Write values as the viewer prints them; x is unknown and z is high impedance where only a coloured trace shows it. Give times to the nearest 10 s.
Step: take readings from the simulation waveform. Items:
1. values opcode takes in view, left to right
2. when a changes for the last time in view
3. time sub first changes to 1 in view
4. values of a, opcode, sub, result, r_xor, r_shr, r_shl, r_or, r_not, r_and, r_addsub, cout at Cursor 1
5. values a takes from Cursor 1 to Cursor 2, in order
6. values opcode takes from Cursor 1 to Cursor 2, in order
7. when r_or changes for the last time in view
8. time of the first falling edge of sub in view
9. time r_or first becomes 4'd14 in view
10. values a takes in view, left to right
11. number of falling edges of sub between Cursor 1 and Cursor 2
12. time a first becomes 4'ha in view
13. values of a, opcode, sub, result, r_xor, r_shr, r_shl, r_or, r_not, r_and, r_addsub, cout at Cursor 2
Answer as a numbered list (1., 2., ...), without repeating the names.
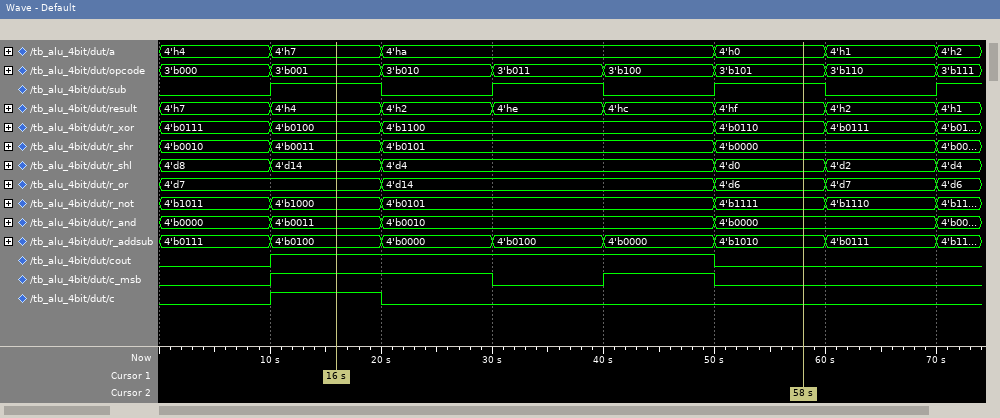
1. 3'b000, 3'b001, 3'b010, 3'b011, 3'b100, 3'b101, 3'b110, 3'b111
2. 70 s
3. 10 s
4. a=4'h7, opcode=3'b001, sub=1, result=4'h4, r_xor=4'b0100, r_shr=4'b0011, r_shl=4'd14, r_or=4'd7, r_not=4'b1000, r_and=4'b0011, r_addsub=4'b0100, cout=1
5. 4'h7, 4'ha, 4'h0
6. 3'b001, 3'b010, 3'b011, 3'b100, 3'b101
7. 70 s
8. 20 s
9. 20 s
10. 4'h4, 4'h7, 4'ha, 4'h0, 4'h1, 4'h2
11. 2
12. 20 s
13. a=4'h0, opcode=3'b101, sub=1, result=4'hf, r_xor=4'b0110, r_shr=4'b0000, r_shl=4'd0, r_or=4'd6, r_not=4'b1111, r_and=4'b0000, r_addsub=4'b1010, cout=0
